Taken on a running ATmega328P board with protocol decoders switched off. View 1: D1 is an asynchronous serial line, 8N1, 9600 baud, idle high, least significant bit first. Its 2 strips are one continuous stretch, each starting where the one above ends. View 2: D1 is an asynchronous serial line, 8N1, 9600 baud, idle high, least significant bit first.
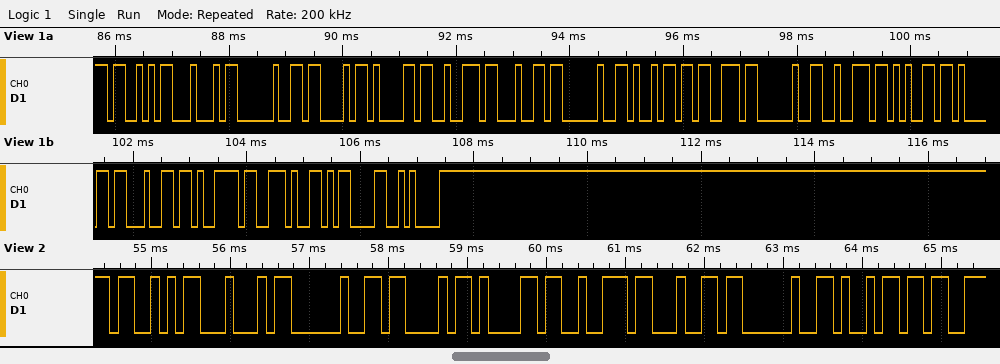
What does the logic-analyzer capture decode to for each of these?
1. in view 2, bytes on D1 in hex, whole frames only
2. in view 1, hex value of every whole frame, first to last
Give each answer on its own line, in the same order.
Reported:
53 44 20 43 61 72 64 20 69
53 44 20 43 61 72 64 20 69 73 20 72 65 61 64 79 2E 0D 0A
